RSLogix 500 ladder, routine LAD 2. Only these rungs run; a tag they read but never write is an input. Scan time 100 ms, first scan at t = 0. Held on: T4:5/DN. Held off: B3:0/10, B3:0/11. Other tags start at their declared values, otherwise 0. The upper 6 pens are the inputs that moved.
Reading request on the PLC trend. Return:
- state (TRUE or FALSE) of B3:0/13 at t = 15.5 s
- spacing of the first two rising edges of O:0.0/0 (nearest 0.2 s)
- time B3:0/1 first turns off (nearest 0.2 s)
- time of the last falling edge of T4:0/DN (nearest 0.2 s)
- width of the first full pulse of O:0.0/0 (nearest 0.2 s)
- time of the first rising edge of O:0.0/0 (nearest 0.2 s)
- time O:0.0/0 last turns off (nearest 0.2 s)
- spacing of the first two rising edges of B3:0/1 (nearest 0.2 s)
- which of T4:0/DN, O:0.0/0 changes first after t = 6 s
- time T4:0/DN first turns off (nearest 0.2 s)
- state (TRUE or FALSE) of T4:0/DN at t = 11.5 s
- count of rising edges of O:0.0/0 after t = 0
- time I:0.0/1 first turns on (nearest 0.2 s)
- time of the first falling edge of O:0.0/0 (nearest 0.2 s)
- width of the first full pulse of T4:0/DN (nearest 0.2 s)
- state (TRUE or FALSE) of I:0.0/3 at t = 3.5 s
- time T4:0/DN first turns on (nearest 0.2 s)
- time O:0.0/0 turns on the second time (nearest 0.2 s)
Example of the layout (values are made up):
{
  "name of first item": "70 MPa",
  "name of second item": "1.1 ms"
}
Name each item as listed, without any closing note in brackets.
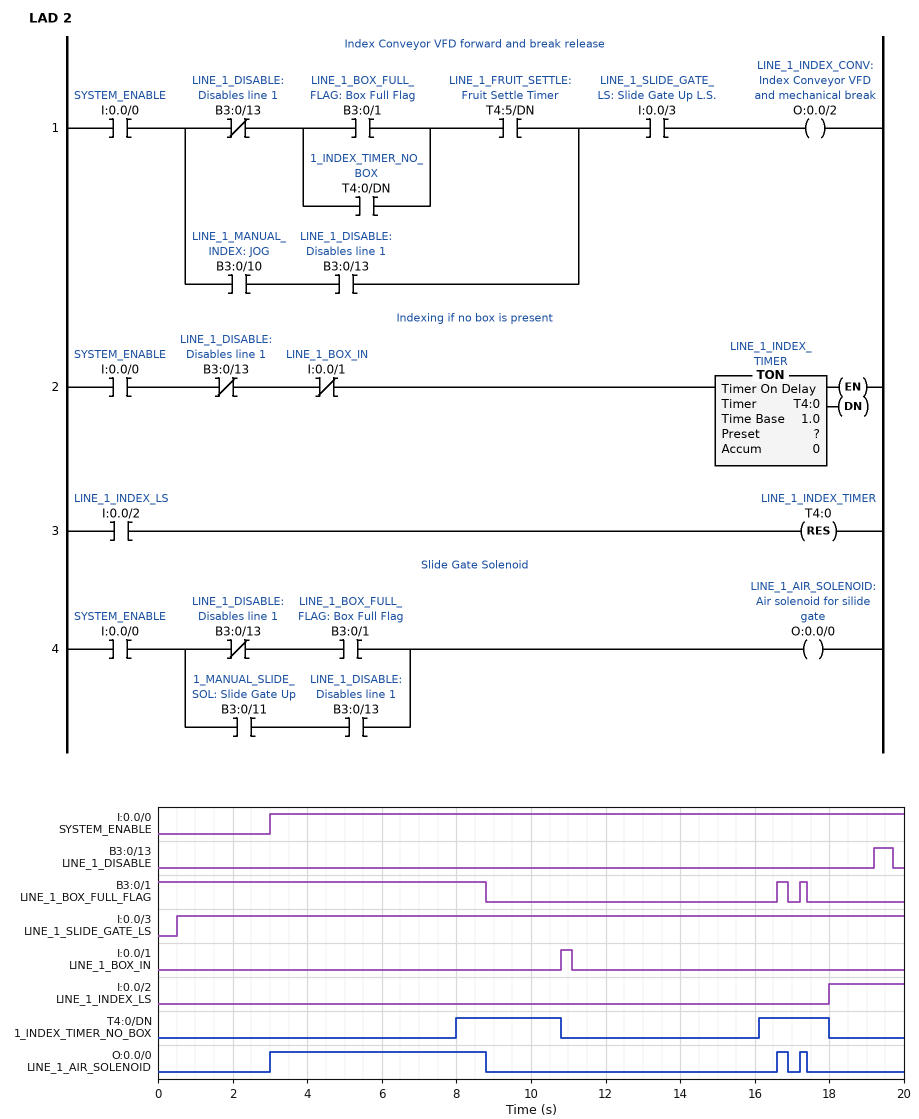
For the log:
{
  "state (TRUE or FALSE) of B3:0/13 at t = 15.5 s": "FALSE",
  "spacing of the first two rising edges of O:0.0/0": "13.6 s",
  "time B3:0/1 first turns off": "8.8 s",
  "time of the last falling edge of T4:0/DN": "18.0 s",
  "width of the first full pulse of O:0.0/0": "5.8 s",
  "time of the first rising edge of O:0.0/0": "3.0 s",
  "time O:0.0/0 last turns off": "17.4 s",
  "spacing of the first two rising edges of B3:0/1": "0.6 s",
  "which of T4:0/DN, O:0.0/0 changes first after t = 6 s": "T4:0/DN",
  "time T4:0/DN first turns off": "10.8 s",
  "state (TRUE or FALSE) of T4:0/DN at t = 11.5 s": "FALSE",
  "count of rising edges of O:0.0/0 after t = 0": "3",
  "time I:0.0/1 first turns on": "10.8 s",
  "time of the first falling edge of O:0.0/0": "8.8 s",
  "width of the first full pulse of T4:0/DN": "2.8 s",
  "state (TRUE or FALSE) of I:0.0/3 at t = 3.5 s": "TRUE",
  "time T4:0/DN first turns on": "8.0 s",
  "time O:0.0/0 turns on the second time": "16.6 s"
}
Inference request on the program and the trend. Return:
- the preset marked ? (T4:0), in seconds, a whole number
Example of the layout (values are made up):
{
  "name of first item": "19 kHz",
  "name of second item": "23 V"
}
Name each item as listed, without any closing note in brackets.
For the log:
{
  "the preset marked ? (T4:0), in seconds, a whole number": "5 s"
}
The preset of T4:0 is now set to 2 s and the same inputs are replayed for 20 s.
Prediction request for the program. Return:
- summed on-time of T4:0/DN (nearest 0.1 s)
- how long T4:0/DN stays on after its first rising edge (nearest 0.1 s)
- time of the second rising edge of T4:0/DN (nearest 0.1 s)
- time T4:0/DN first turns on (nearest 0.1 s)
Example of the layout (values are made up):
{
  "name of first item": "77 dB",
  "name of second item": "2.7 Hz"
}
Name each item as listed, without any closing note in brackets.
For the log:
{
  "summed on-time of T4:0/DN": "10.7 s",
  "how long T4:0/DN stays on after its first rising edge": "5.8 s",
  "time of the second rising edge of T4:0/DN": "13.1 s",
  "time T4:0/DN first turns on": "5.0 s"
}
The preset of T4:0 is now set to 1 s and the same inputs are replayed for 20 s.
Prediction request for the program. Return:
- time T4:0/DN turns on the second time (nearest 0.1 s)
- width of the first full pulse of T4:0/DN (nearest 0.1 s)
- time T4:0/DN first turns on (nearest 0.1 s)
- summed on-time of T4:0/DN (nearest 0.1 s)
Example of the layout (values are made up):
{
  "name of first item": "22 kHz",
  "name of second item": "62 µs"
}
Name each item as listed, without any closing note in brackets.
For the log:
{
  "time T4:0/DN turns on the second time": "12.1 s",
  "width of the first full pulse of T4:0/DN": "6.8 s",
  "time T4:0/DN first turns on": "4.0 s",
  "summed on-time of T4:0/DN": "12.7 s"
}
